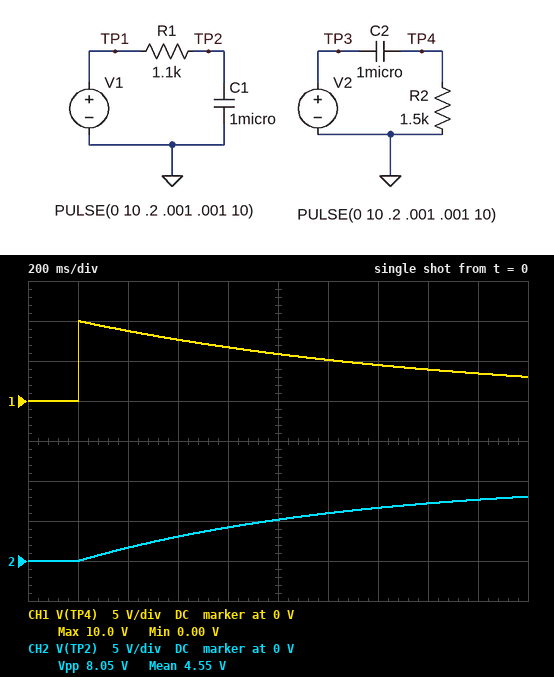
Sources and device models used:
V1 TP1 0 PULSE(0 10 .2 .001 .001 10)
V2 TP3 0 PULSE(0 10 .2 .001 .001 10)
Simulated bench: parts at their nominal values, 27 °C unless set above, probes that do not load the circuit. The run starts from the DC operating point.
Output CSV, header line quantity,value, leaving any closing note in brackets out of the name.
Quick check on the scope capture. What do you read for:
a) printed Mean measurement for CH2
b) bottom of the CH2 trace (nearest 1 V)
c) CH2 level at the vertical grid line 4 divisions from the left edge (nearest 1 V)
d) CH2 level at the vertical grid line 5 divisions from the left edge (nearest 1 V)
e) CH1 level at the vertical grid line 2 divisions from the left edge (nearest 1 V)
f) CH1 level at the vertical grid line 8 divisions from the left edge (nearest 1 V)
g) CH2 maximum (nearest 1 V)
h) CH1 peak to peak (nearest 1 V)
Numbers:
quantity,value
printed Mean measurement for CH2,4.55 V
bottom of the CH2 trace,0 V
CH2 level at the vertical grid line 4 divisions from the left edge,4 V
CH2 level at the vertical grid line 5 divisions from the left edge,5 V
CH1 level at the vertical grid line 2 divisions from the left edge,9 V
CH1 level at the vertical grid line 8 divisions from the left edge,4 V
CH2 maximum,8 V
CH1 peak to peak,10 V
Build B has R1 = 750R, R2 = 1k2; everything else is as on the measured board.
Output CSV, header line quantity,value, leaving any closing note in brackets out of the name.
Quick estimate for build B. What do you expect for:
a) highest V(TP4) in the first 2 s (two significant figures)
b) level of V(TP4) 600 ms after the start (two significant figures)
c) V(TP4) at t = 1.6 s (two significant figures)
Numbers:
quantity,value
highest V(TP4) in the first 2 s,10 V
level of V(TP4) 600 ms after the start,7.2 V
V(TP4) at t = 1.6 s,3.1 V
